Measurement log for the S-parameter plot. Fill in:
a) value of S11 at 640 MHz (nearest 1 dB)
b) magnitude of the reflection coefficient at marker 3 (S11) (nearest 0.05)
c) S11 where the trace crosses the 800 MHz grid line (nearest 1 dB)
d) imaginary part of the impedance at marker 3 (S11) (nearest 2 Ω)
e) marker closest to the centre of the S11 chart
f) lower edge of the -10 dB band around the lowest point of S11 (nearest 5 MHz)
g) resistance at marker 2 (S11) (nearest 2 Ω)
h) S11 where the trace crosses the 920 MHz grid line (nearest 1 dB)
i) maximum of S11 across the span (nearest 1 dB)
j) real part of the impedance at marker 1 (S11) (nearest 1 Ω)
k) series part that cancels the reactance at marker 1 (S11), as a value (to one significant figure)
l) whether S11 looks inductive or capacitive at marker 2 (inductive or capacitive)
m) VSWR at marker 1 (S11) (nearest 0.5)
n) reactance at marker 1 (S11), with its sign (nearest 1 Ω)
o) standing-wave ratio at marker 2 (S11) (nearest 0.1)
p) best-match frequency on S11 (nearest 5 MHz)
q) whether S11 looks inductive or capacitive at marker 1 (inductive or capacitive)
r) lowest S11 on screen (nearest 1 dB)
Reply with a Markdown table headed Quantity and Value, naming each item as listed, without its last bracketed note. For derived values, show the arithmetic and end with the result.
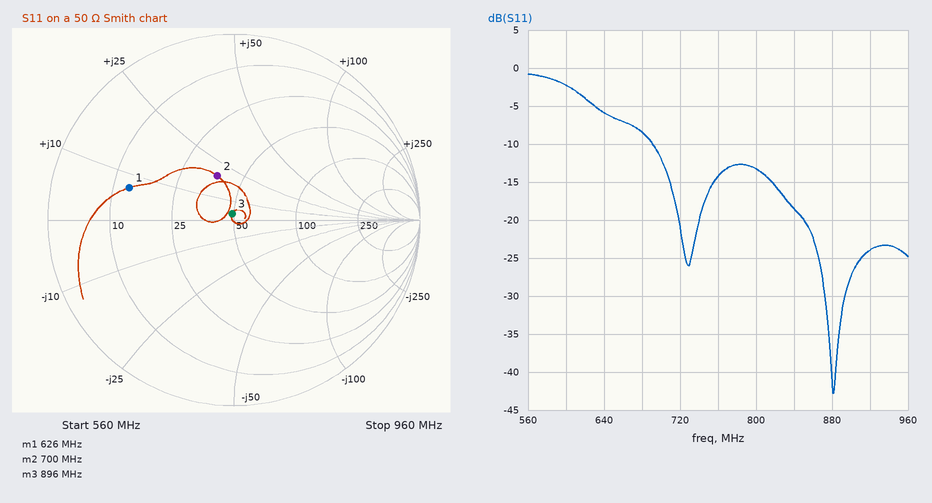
| Quantity | Value |
|---|---|
| value of S11 at 640 MHz | -6 dB |
| magnitude of the reflection coefficient at marker 3 (S11) | 0.05 |
| S11 where the trace crosses the 800 MHz grid line | -13 dB |
| imaginary part of the impedance at marker 3 (S11) | +4 Ω |
| marker closest to the centre of the S11 chart | marker 3 |
| lower edge of the -10 dB band around the lowest point of S11 | 690 MHz |
| resistance at marker 2 (S11) | 38 Ω |
| S11 where the trace crosses the 920 MHz grid line | -24 dB |
| maximum of S11 across the span | -1 dB |
| real part of the impedance at marker 1 (S11) | 13 Ω |
| series part that cancels the reactance at marker 1 (S11), as a value | C = 1/(2π × 626 MHz × 7 Ω) ≈ 36.3 pF, so 40 pF to one significant figure |
| whether S11 looks inductive or capacitive at marker 2 | inductive |
| VSWR at marker 1 (S11) | 4.0 |
| reactance at marker 1 (S11), with its sign | +7 Ω |
| standing-wave ratio at marker 2 (S11) | 1.7 |
| best-match frequency on S11 | 880 MHz |
| whether S11 looks inductive or capacitive at marker 1 | inductive |
| lowest S11 on screen | -43 dB |
